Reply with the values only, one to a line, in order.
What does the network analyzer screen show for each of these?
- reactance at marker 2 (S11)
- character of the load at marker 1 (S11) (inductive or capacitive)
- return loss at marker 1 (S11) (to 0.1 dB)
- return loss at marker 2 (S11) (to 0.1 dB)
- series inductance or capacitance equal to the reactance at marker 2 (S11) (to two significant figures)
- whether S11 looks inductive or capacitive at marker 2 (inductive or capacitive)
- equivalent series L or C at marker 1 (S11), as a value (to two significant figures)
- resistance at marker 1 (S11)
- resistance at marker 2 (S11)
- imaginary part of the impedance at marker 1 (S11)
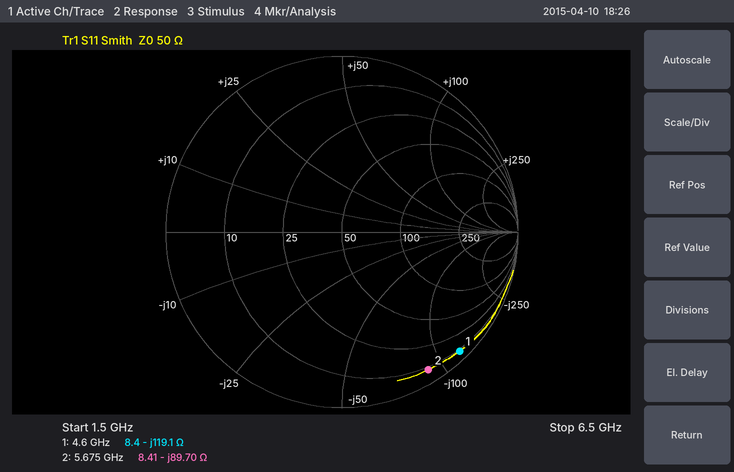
-89.70 Ω
capacitive
0.4 dB
0.7 dB
310 fF
capacitive
290 fF
8.4 Ω
8.41 Ω
-119.1 Ω
